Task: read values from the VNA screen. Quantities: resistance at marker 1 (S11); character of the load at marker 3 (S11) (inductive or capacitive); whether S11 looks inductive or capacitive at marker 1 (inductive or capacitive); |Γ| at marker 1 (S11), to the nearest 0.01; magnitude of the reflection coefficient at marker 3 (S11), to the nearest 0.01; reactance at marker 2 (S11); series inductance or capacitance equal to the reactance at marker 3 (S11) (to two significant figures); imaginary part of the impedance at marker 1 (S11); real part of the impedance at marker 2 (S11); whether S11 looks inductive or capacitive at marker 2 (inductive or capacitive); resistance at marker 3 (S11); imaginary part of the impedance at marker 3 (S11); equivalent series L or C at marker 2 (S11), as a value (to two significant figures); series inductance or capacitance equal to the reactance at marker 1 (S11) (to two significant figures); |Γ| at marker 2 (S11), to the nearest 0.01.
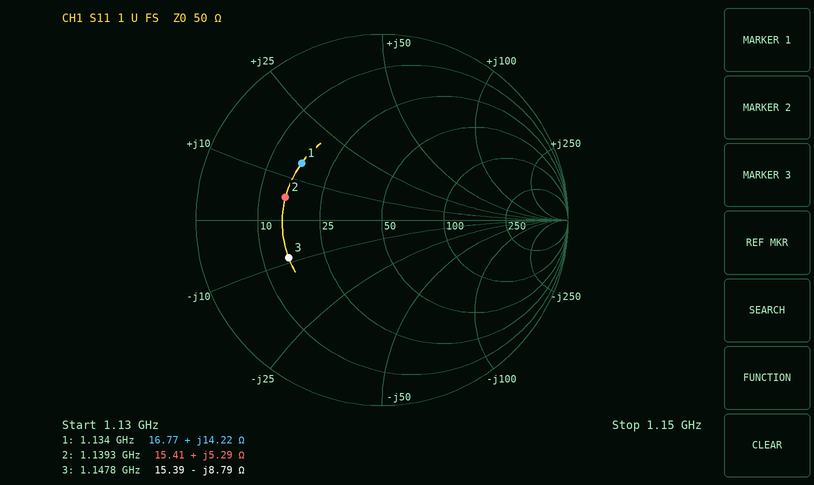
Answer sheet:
16.77 Ω
capacitive
inductive
0.53
0.54
+5.29 Ω
16 pF
+14.22 Ω
15.41 Ω
inductive
15.39 Ω
-8.79 Ω
740 pH
2.0 nH
0.53
